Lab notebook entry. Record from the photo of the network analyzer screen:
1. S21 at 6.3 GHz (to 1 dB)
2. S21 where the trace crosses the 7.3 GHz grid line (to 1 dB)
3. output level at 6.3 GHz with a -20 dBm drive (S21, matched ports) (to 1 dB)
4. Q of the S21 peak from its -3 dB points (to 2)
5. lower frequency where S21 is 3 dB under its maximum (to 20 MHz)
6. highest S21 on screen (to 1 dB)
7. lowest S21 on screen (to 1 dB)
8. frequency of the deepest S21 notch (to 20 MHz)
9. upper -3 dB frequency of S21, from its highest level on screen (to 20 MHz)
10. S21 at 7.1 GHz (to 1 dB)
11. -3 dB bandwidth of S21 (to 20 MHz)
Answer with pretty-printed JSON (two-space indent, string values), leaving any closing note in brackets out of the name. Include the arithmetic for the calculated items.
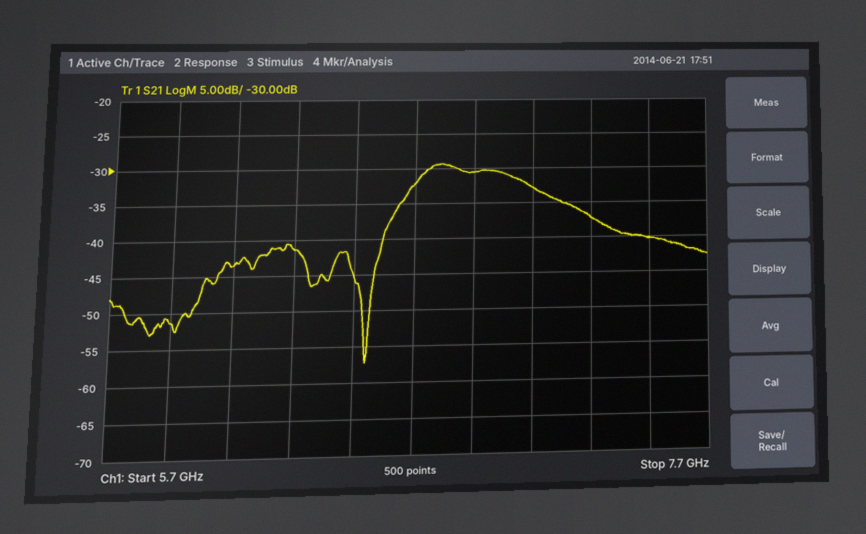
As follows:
{
  "S21 at 6.3 GHz": "-41 dB",
  "S21 where the trace crosses the 7.3 GHz grid line": "-37 dB",
  "output level at 6.3 GHz with a -20 dBm drive (S21, matched ports)": "-20 dBm + (-41 dB) = -61 dBm",
  "Q of the S21 peak from its -3 dB points": "6.89 GHz / 380 MHz ≈ 18",
  "lower frequency where S21 is 3 dB under its maximum": "6.70 GHz",
  "highest S21 on screen": "-29 dB",
  "lowest S21 on screen": "-57 dB",
  "frequency of the deepest S21 notch": "6.54 GHz",
  "upper -3 dB frequency of S21, from its highest level on screen": "7.08 GHz",
  "S21 at 7.1 GHz": "-33 dB",
  "-3 dB bandwidth of S21": "7.08 GHz − 6.70 GHz = 380 MHz"
}
